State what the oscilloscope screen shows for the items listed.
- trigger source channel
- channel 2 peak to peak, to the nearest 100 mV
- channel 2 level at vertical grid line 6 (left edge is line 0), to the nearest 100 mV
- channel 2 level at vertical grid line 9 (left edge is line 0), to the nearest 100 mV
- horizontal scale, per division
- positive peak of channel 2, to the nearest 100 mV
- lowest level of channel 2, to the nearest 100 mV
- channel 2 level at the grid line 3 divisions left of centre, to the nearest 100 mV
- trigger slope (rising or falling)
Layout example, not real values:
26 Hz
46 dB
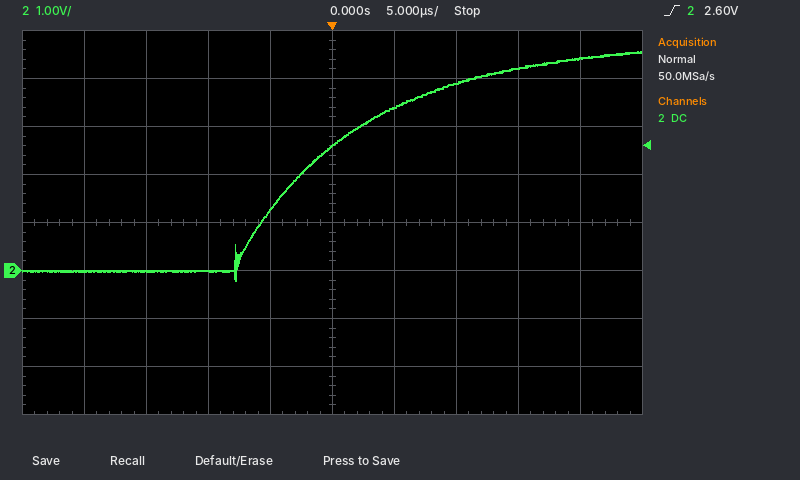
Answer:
channel 2
4.8 V
3.4 V
4.4 V
5 µs
4.6 V
-200 mV
0.0 V
rising
